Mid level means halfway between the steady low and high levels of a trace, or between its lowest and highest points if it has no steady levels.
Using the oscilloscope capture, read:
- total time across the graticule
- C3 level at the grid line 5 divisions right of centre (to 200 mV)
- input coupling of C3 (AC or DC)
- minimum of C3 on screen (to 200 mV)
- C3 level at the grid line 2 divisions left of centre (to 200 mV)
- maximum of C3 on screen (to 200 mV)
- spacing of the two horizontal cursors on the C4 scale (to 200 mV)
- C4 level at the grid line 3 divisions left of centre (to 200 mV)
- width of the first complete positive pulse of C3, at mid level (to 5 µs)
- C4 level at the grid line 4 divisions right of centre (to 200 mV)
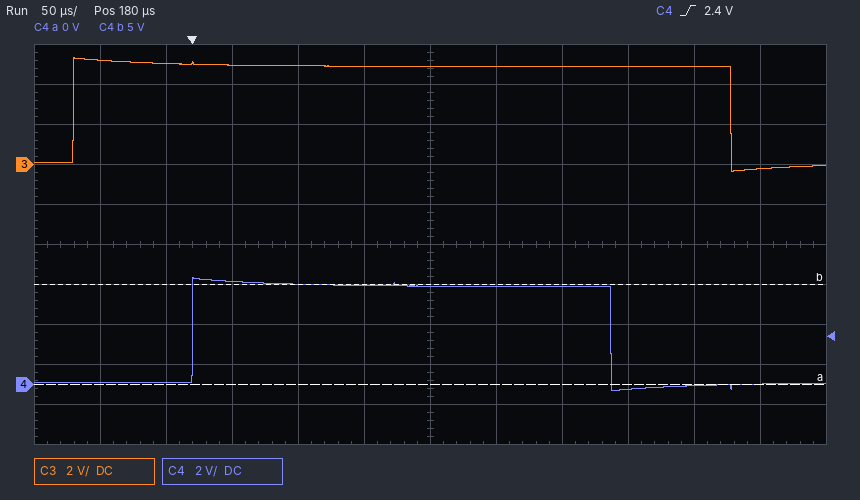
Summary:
600 µs
-200 mV
DC
-400 mV
5.0 V
5.4 V
5.0 V
5.2 V
500 µs
0.0 V
